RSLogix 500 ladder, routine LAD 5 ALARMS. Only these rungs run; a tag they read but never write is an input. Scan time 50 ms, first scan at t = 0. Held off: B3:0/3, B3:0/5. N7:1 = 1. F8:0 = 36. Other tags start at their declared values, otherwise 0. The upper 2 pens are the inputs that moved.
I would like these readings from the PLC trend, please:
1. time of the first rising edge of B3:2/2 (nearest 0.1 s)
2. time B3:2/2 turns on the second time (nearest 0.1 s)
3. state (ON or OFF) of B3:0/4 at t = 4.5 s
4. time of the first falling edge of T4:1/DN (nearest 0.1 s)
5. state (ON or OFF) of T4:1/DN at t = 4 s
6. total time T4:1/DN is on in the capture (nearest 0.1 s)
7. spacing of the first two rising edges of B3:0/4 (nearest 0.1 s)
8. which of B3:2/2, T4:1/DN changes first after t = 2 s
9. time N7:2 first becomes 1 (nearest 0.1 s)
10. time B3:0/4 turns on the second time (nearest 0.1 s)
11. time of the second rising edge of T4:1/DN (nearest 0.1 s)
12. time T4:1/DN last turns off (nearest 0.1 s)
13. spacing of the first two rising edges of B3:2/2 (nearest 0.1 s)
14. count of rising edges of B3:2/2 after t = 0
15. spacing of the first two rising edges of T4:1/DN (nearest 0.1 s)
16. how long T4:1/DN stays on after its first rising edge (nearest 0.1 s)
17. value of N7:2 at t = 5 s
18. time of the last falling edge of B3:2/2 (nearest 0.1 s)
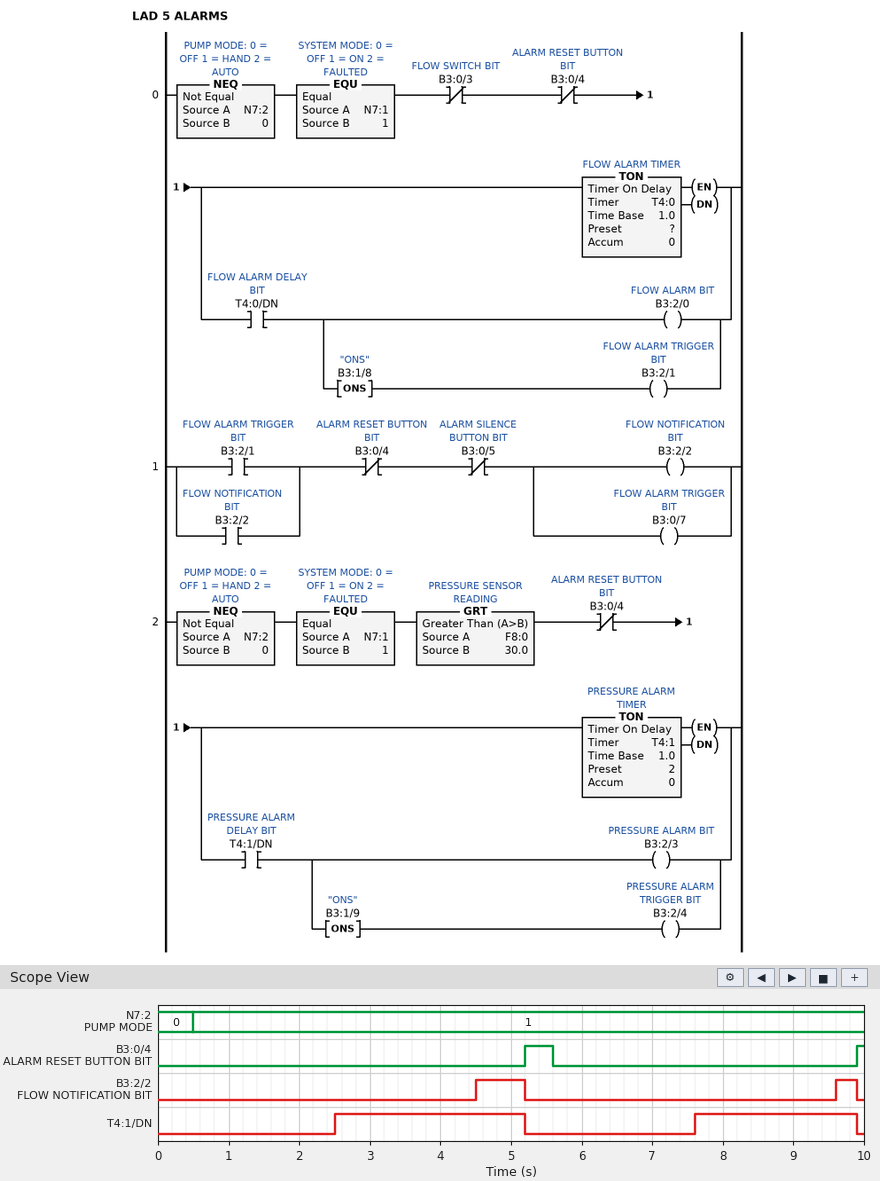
4.5 s
9.6 s
OFF
5.2 s
ON
5.0 s
4.7 s
T4:1/DN
0.5 s
9.9 s
7.6 s
9.9 s
5.1 s
2
5.1 s
2.7 s
1
9.9 s
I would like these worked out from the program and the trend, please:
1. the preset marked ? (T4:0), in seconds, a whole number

4 s
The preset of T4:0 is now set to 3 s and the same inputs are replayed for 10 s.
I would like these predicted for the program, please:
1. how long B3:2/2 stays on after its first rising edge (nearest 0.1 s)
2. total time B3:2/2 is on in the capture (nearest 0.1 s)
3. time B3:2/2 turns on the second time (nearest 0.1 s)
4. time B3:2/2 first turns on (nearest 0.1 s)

1.7 s
3.0 s
8.6 s
3.5 s
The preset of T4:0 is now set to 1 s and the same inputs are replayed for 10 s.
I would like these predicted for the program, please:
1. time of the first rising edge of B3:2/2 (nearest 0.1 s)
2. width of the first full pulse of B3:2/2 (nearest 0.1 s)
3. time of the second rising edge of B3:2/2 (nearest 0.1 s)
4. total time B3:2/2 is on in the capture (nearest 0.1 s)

1.5 s
3.7 s
6.6 s
7.0 s
